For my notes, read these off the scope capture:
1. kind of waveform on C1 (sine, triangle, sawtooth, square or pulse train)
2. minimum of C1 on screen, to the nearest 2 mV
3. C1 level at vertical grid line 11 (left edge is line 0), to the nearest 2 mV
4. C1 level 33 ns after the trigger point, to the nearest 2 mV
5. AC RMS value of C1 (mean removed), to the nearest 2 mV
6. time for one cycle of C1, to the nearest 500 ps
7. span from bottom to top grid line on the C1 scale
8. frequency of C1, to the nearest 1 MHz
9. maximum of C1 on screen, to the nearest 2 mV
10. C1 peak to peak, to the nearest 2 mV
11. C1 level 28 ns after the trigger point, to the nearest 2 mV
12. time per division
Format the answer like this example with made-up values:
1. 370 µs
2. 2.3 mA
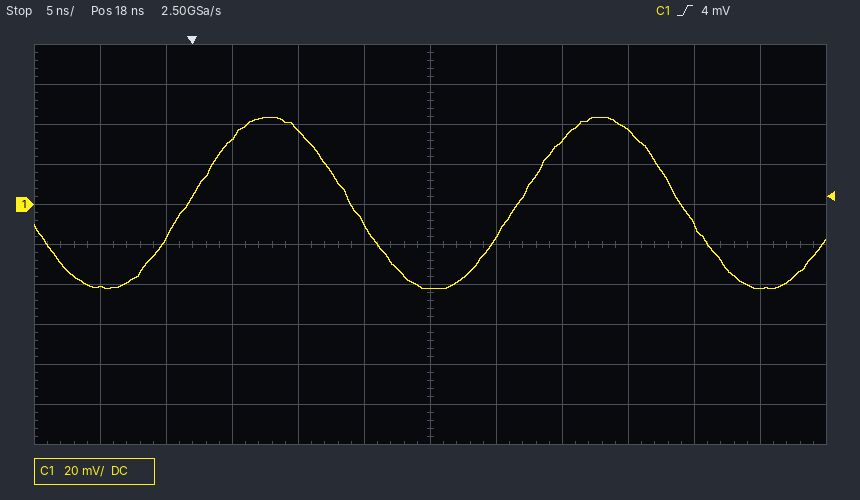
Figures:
1. sine
2. -42 mV
3. -42 mV
4. 38 mV
5. 30 mV
6. 25.0 ns
7. 200 mV
8. 40 MHz
9. 44 mV
10. 86 mV
11. 32 mV
12. 5 ns
